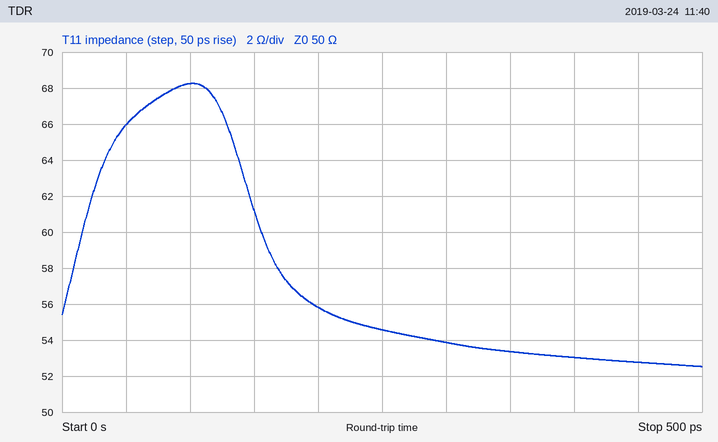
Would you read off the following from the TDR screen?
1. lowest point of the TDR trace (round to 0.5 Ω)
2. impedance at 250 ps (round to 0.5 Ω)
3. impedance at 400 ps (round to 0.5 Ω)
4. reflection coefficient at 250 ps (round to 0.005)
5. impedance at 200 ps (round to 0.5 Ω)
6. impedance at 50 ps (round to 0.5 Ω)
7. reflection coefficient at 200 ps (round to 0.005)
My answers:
52.5 Ω
54.5 Ω
53.0 Ω
+0.045
56.0 Ω
66.0 Ω
+0.055
